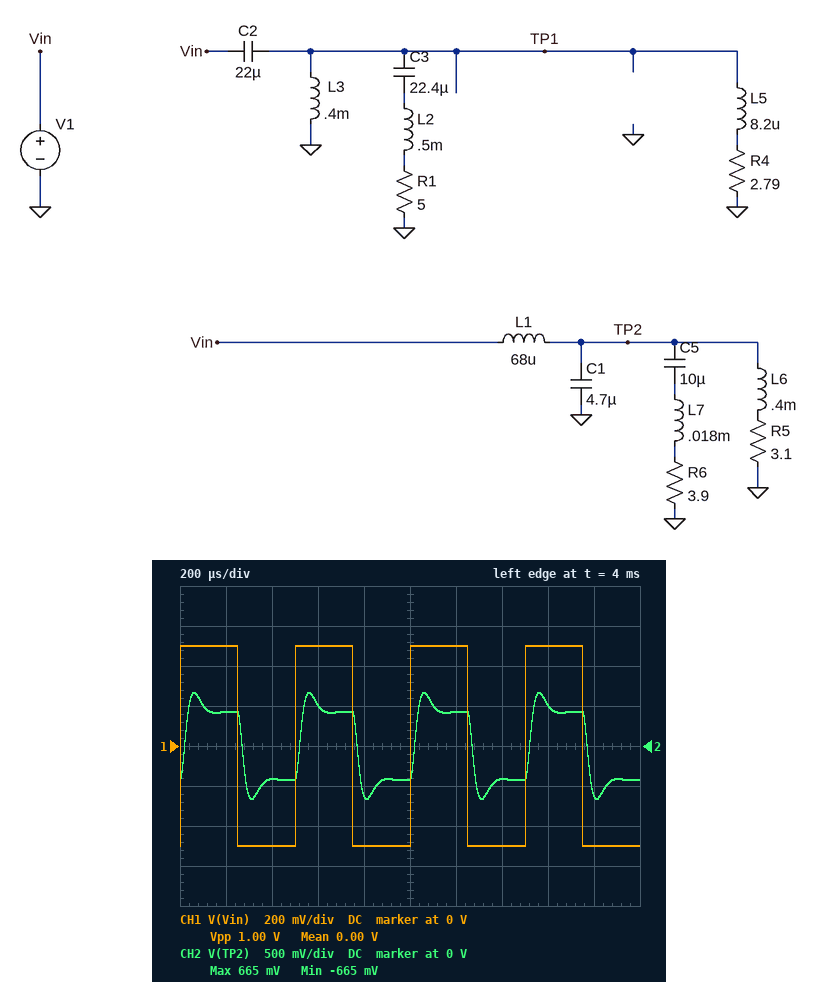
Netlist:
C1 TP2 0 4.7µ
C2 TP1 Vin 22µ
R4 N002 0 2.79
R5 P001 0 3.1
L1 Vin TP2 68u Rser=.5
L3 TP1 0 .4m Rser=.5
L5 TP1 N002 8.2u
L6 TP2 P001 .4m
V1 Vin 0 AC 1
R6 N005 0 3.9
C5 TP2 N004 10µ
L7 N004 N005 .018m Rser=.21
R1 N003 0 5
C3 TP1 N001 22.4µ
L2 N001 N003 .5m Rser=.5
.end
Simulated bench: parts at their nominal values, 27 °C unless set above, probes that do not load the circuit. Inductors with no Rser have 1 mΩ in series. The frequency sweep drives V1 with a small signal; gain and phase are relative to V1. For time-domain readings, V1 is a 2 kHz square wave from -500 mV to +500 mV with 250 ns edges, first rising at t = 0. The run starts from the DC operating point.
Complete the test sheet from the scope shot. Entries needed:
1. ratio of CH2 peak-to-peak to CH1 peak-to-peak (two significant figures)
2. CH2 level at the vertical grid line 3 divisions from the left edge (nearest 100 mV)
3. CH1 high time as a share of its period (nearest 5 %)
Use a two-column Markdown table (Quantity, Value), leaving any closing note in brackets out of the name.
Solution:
| Quantity | Value |
|---|---|
| ratio of CH2 peak-to-peak to CH1 peak-to-peak | 1.3 |
| CH2 level at the vertical grid line 3 divisions from the left edge | 500 mV |
| CH1 high time as a share of its period | 50 % |
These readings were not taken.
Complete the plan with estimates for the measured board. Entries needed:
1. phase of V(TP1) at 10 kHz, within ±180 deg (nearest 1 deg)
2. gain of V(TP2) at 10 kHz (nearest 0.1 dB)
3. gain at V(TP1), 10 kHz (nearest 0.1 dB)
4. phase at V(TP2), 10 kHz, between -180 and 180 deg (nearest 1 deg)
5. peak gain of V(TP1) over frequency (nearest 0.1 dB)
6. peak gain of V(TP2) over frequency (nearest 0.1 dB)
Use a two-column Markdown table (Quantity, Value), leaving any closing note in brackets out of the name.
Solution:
| Quantity | Value |
|---|---|
| phase of V(TP1) at 10 kHz, within ±180 deg | 16 deg |
| gain of V(TP2) at 10 kHz | -1.5 dB |
| gain at V(TP1), 10 kHz | 0.6 dB |
| phase at V(TP2), 10 kHz, between -180 and 180 deg | -94 deg |
| peak gain of V(TP1) over frequency | 0.7 dB |
| peak gain of V(TP2) over frequency | 1.3 dB |
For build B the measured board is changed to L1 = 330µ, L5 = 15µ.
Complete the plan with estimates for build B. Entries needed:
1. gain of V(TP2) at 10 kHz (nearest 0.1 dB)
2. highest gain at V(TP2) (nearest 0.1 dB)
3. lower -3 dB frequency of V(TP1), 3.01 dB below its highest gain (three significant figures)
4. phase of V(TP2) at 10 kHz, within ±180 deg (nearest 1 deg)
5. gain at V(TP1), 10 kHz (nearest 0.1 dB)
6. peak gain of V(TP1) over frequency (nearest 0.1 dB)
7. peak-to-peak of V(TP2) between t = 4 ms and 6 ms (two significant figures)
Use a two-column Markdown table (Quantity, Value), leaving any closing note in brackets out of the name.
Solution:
| Quantity | Value |
|---|---|
| gain of V(TP2) at 10 kHz | -17.0 dB |
| highest gain at V(TP2) | -0.5 dB |
| lower -3 dB frequency of V(TP1), 3.01 dB below its highest gain | 2.67 kHz |
| phase of V(TP2) at 10 kHz, within ±180 deg | -132 deg |
| gain at V(TP1), 10 kHz | 0.9 dB |
| peak gain of V(TP1) over frequency | 1.0 dB |
| peak-to-peak of V(TP2) between t = 4 ms and 6 ms | 1.0 V |
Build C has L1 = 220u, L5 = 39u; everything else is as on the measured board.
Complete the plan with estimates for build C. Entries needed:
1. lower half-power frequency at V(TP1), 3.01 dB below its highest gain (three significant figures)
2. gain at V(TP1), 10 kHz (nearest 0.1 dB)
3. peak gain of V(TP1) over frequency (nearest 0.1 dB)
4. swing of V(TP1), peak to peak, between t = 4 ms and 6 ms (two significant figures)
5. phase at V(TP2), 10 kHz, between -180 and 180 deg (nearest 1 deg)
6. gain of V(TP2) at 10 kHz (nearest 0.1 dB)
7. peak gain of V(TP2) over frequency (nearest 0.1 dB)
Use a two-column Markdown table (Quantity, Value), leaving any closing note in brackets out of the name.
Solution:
| Quantity | Value |
|---|---|
| lower half-power frequency at V(TP1), 3.01 dB below its highest gain | 2.87 kHz |
| gain at V(TP1), 10 kHz | 1.6 dB |
| peak gain of V(TP1) over frequency | 2.3 dB |
| swing of V(TP1), peak to peak, between t = 4 ms and 6 ms | 2.0 V |
| phase at V(TP2), 10 kHz, between -180 and 180 deg | -128 deg |
| gain of V(TP2) at 10 kHz | -13.1 dB |
| peak gain of V(TP2) over frequency | 0.6 dB |
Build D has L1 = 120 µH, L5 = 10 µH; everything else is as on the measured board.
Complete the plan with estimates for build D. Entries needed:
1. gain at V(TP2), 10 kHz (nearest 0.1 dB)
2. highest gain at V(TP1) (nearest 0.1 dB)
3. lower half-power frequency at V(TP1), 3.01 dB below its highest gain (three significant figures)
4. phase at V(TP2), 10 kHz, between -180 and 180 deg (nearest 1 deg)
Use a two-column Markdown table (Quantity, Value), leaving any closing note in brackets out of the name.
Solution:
| Quantity | Value |
|---|---|
| gain at V(TP2), 10 kHz | -7.0 dB |
| highest gain at V(TP1) | 0.8 dB |
| lower half-power frequency at V(TP1), 3.01 dB below its highest gain | 2.62 kHz |
| phase at V(TP2), 10 kHz, between -180 and 180 deg | -117 deg |
